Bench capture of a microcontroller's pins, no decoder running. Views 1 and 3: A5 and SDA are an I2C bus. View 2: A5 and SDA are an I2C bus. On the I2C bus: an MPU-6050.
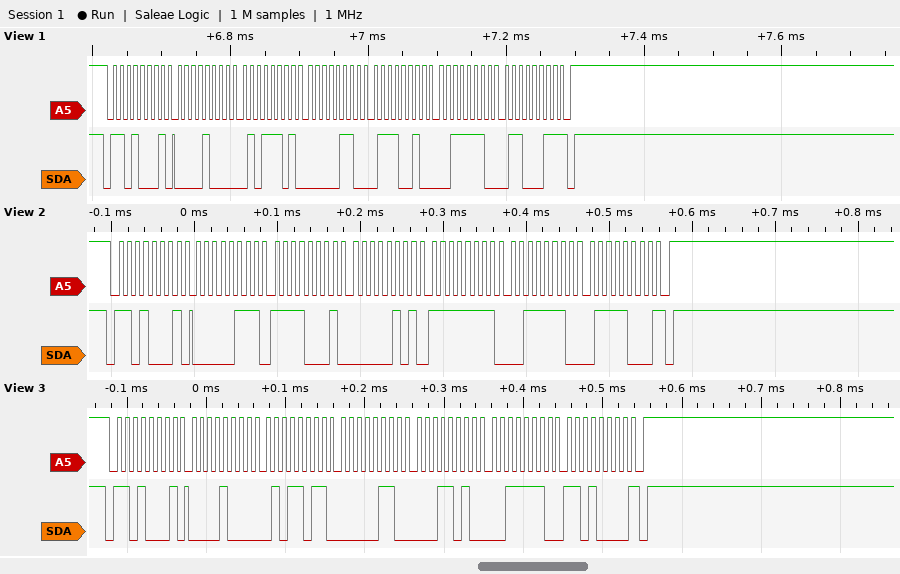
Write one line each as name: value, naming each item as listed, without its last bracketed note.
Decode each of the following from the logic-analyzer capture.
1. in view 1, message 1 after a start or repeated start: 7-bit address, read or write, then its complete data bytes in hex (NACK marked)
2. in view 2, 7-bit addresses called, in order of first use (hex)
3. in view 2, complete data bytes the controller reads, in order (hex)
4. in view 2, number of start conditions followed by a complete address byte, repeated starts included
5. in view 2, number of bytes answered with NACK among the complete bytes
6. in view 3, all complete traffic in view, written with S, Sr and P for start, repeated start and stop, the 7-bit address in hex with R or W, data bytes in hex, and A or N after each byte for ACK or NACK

in view 1, message 1 after a start or repeated start: 7-bit address, read or write, then its complete data bytes in hex: 0x68 read: 08 5D 06 72 3E 63 NACK
in view 2, 7-bit addresses called, in order of first use: 0x68
in view 2, complete data bytes the controller reads, in order: 07 F1 05 FF 3E 78
in view 2, number of start conditions followed by a complete address byte, repeated starts included: 1
in view 2, number of bytes answered with NACK among the complete bytes: 1
in view 3, all complete traffic in view, written with S, Sr and P for start, repeated start and stop, the 7-bit address in hex with R or W, data bytes in hex, and A or N after each byte for ACK or NACK: S 68R A 08 A 5B A 06 A 1A A 3E A D0 N P
